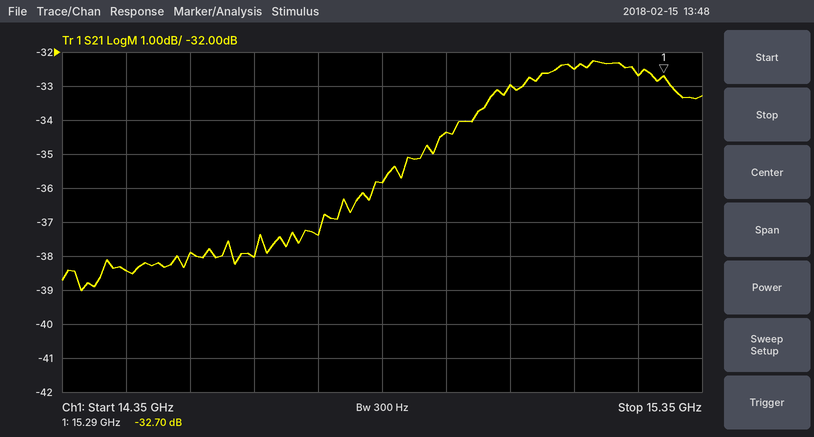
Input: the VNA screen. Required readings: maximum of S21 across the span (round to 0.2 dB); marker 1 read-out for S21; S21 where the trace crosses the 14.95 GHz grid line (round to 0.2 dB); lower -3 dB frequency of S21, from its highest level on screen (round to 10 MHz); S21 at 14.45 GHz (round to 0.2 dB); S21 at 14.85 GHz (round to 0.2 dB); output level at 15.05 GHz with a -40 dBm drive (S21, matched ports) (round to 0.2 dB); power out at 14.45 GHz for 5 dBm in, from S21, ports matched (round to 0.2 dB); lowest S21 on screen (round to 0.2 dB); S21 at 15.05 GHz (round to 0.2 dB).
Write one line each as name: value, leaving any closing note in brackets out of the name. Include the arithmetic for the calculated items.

maximum of S21 across the span: -32.2 dB
marker 1 read-out for S21: -32.70 dB
S21 where the trace crosses the 14.95 GHz grid line: -34.4 dB
lower -3 dB frequency of S21, from its highest level on screen: 14.89 GHz
S21 at 14.45 GHz: -38.4 dB
S21 at 14.85 GHz: -35.8 dB
output level at 15.05 GHz with a -40 dBm drive (S21, matched ports): -40 dBm + (-33.0 dB) = -73.0 dBm
power out at 14.45 GHz for 5 dBm in, from S21, ports matched: 5 dBm + (-38.4 dB) = -33.4 dBm
lowest S21 on screen: -39.0 dB
S21 at 15.05 GHz: -33.0 dB
